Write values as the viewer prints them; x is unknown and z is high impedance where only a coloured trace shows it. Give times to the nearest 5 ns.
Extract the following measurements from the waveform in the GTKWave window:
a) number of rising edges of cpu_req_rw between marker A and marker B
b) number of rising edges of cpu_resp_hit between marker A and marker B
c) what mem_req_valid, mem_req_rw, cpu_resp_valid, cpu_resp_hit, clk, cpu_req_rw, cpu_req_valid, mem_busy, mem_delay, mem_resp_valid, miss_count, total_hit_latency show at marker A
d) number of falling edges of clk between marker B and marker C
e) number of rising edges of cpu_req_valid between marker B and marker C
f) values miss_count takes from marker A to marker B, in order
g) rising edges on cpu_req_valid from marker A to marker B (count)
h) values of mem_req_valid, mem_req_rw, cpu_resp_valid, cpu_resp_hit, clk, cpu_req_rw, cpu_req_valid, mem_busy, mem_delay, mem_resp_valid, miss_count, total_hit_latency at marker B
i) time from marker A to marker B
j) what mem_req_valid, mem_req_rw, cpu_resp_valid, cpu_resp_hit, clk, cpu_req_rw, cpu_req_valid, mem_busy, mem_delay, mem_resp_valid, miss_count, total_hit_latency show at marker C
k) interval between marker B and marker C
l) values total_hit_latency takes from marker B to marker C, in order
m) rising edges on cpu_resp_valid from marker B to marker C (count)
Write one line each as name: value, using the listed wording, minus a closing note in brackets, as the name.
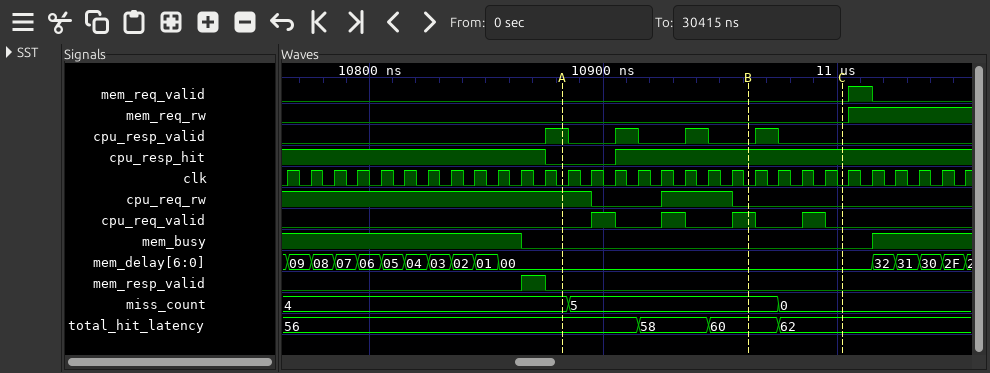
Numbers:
number of rising edges of cpu_req_rw between marker A and marker B: 1
number of rising edges of cpu_resp_hit between marker A and marker B: 1
what mem_req_valid, mem_req_rw, cpu_resp_valid, cpu_resp_hit, clk, cpu_req_rw, cpu_req_valid, mem_busy, mem_delay, mem_resp_valid, miss_count, total_hit_latency show at marker A: mem_req_valid=0, mem_req_rw=0, cpu_resp_valid=1, cpu_resp_hit=0, clk=0, cpu_req_rw=1, cpu_req_valid=0, mem_busy=0, mem_delay=00, mem_resp_valid=0, miss_count=4, total_hit_latency=56
number of falling edges of clk between marker B and marker C: 4
number of rising edges of cpu_req_valid between marker B and marker C: 1
values miss_count takes from marker A to marker B, in order: 4, 5
rising edges on cpu_req_valid from marker A to marker B: 3
values of mem_req_valid, mem_req_rw, cpu_resp_valid, cpu_resp_hit, clk, cpu_req_rw, cpu_req_valid, mem_busy, mem_delay, mem_resp_valid, miss_count, total_hit_latency at marker B: mem_req_valid=0, mem_req_rw=0, cpu_resp_valid=0, cpu_resp_hit=1, clk=0, cpu_req_rw=0, cpu_req_valid=1, mem_busy=0, mem_delay=00, mem_resp_valid=0, miss_count=5, total_hit_latency=60
time from marker A to marker B: 80 ns
what mem_req_valid, mem_req_rw, cpu_resp_valid, cpu_resp_hit, clk, cpu_req_rw, cpu_req_valid, mem_busy, mem_delay, mem_resp_valid, miss_count, total_hit_latency show at marker C: mem_req_valid=0, mem_req_rw=0, cpu_resp_valid=0, cpu_resp_hit=1, clk=0, cpu_req_rw=0, cpu_req_valid=0, mem_busy=0, mem_delay=00, mem_resp_valid=0, miss_count=0, total_hit_latency=62
interval between marker B and marker C: 40 ns
values total_hit_latency takes from marker B to marker C, in order: 60, 62
rising edges on cpu_resp_valid from marker B to marker C: 1
